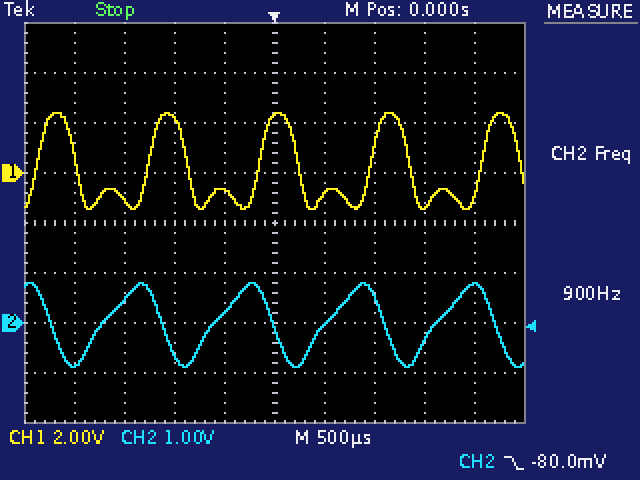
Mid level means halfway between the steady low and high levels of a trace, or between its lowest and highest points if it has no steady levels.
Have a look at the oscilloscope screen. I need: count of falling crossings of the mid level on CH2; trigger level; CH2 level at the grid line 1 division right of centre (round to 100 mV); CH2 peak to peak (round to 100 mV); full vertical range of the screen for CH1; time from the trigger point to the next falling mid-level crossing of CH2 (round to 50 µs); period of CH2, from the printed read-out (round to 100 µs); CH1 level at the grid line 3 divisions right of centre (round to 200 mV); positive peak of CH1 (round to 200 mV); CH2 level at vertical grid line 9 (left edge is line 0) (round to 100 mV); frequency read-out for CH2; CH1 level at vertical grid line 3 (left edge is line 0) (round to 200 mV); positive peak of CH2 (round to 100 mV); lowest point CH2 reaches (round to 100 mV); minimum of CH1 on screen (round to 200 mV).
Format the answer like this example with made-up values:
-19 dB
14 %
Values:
5
-80.0 mV
0.0 V
1.7 V
16 V
1.10 ms
1.1 ms
-1.4 V
2.4 V
800 mV
900 Hz
2.2 V
800 mV
-900 mV
-1.4 V
